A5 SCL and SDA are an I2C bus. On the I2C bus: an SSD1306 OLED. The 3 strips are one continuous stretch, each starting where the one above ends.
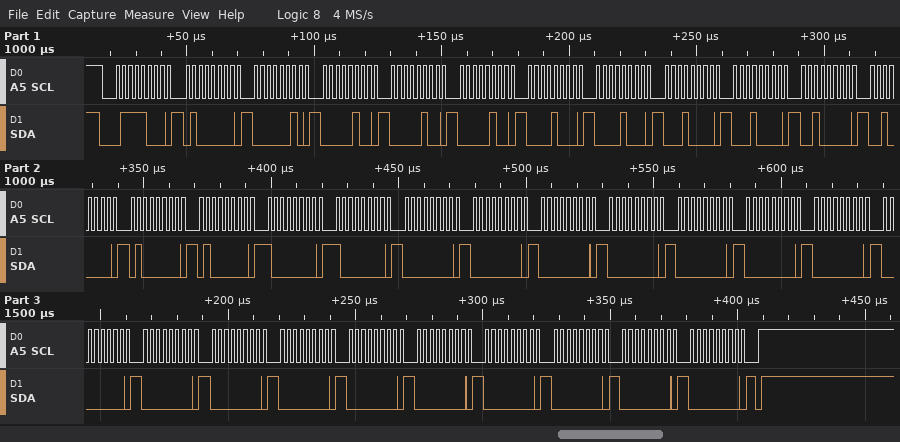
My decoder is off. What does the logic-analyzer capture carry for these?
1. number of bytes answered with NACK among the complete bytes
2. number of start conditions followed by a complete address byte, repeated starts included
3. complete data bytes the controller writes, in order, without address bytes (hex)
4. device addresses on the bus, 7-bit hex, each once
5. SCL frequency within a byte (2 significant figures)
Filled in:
0
1
40 02 04 04 04 08 08 10 10 20 20 40 40 80 80 00 00 00 00 00 00 00 00 00 00 00 00 00 00 00 00 00
0x3C
400 kHz
